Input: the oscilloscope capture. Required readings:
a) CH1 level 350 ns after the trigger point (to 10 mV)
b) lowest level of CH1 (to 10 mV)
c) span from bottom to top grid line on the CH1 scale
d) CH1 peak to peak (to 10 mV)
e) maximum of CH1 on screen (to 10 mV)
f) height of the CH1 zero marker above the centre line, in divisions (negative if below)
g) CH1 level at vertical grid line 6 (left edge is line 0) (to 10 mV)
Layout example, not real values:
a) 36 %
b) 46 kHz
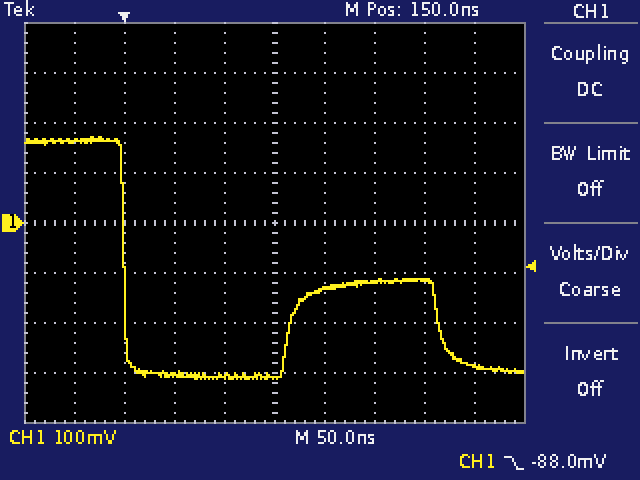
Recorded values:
a) -290 mV
b) -310 mV
c) 800 mV
d) 480 mV
e) 170 mV
f) 0.0 div
g) -130 mV
